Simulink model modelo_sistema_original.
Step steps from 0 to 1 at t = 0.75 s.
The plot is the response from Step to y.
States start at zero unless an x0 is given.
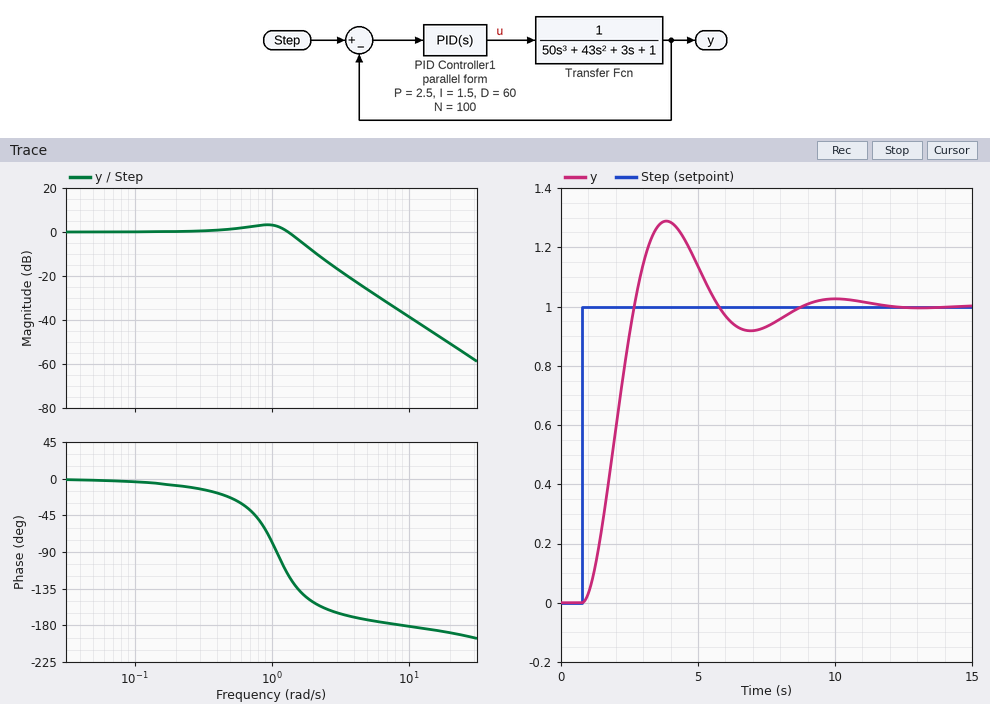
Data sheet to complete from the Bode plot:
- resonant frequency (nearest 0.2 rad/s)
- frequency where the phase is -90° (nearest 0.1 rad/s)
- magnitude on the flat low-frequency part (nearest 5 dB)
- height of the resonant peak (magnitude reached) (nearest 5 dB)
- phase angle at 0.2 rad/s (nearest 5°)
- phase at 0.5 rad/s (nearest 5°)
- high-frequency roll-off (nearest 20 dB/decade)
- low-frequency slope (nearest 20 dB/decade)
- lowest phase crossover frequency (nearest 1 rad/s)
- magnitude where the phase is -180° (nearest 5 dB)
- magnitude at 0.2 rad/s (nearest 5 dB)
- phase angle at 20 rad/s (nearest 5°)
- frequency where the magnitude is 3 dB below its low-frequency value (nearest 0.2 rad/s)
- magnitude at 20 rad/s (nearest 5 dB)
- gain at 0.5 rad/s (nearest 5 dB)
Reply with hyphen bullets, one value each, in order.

- 1.0 rad/s
- 1.1 rad/s
- 0 dB
- 5 dB
- -10°
- -25°
- -40 dB/decade
- 0 dB/decade
- 9 rad/s
- -35 dB
- 0 dB
- -190°
- 1.6 rad/s
- -50 dB
- 0 dB
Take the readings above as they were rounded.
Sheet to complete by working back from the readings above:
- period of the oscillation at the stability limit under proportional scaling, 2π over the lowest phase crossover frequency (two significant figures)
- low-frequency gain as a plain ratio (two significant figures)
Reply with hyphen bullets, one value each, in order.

- 0.70 s
- 1.0
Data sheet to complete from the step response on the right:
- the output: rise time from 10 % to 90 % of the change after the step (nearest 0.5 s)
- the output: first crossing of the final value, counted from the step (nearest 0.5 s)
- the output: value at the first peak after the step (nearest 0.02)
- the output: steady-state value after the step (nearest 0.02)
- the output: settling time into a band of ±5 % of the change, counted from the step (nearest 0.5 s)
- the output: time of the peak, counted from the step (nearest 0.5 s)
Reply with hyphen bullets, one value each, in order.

- 1.5 s
- 2.0 s
- 1.28
- 1.00
- 7.0 s
- 3.0 s
